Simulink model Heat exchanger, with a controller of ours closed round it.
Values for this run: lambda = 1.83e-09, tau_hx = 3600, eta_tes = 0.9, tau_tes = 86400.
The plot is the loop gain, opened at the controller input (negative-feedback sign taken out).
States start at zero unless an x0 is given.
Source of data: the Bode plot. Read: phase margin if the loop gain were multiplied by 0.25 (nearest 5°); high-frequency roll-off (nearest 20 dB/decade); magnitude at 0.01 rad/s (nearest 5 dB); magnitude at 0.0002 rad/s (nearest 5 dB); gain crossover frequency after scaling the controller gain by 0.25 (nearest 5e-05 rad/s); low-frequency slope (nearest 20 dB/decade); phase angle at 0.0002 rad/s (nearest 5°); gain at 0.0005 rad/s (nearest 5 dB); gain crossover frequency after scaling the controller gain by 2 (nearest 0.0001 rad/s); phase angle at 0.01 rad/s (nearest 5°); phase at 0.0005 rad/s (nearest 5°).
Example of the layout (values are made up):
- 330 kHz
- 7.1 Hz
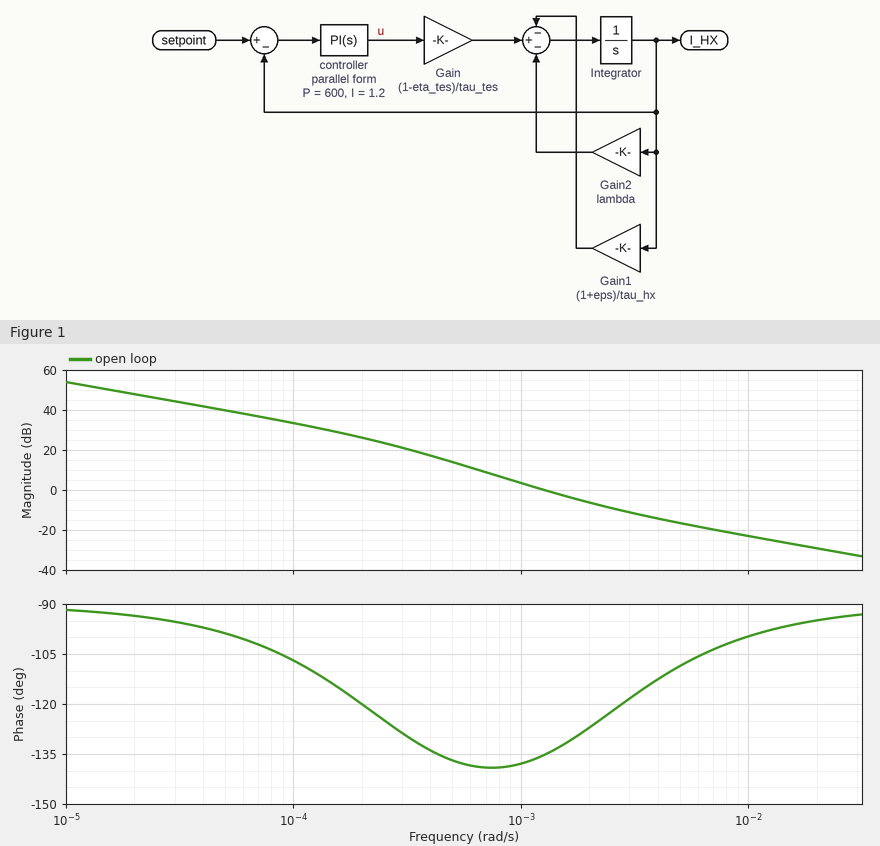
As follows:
- 40°
- -20 dB/decade
- -25 dB
- 25 dB
- 0.00055 rad/s
- -20 dB/decade
- -120°
- 15 dB
- 0.0020 rad/s
- -100°
- -135°
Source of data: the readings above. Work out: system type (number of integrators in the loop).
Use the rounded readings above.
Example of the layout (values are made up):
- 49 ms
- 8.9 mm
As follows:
- 1
